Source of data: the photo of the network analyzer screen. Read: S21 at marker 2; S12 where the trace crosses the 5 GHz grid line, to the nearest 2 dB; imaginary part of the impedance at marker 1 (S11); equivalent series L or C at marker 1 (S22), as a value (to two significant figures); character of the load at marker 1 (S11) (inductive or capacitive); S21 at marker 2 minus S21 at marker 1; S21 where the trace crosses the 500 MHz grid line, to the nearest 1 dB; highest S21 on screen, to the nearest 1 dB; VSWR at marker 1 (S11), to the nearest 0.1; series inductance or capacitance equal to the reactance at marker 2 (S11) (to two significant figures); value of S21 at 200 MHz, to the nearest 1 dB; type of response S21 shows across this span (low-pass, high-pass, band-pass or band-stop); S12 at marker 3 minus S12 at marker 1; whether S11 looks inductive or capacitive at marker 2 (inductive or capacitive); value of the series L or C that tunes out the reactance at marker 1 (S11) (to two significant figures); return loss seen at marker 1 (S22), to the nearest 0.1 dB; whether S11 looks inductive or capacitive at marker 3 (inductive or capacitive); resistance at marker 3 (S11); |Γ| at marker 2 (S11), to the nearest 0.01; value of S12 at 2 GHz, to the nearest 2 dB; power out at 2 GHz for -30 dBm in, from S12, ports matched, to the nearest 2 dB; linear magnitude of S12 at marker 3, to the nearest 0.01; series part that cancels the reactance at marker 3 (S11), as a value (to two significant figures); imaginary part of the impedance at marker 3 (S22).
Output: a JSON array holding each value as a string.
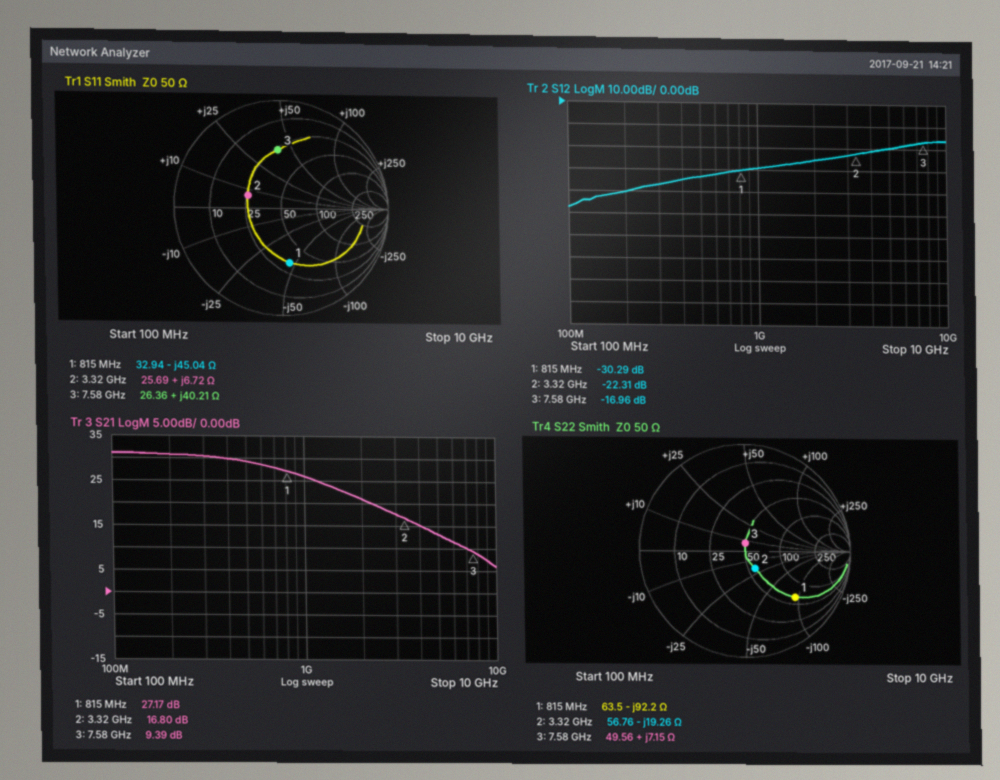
["16.80 dB", "-20 dB", "-45.04 Ω", "2.1 pF", "capacitive", "-10.37 dB", "29 dB", "31 dB", "3.1", "320 pH", "31 dB", "low-pass", "13.33 dB", "inductive", "8.8 nH", "3.9 dB", "inductive", "26.36 Ω", "0.33", "-26 dB", "-56 dBm", "0.14", "520 fF", "+7.15 Ω"]
